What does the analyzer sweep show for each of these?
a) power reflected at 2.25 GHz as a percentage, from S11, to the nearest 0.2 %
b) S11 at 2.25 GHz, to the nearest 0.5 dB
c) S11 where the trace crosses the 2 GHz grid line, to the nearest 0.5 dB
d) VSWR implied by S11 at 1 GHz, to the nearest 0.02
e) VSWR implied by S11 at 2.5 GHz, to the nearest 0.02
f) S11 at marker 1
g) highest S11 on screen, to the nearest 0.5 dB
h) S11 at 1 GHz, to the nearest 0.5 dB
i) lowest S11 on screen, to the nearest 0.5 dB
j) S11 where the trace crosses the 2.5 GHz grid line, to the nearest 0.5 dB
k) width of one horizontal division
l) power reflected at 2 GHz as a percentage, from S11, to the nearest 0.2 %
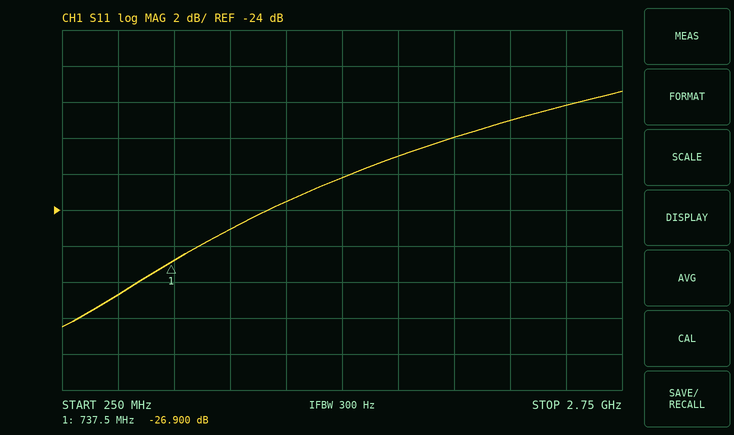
1.2 %
-19.0 dB
-20.0 dB
1.12
1.28
-26.900 dB
-17.5 dB
-25.0 dB
-30.5 dB
-18.0 dB
250 MHz
1.0 %
